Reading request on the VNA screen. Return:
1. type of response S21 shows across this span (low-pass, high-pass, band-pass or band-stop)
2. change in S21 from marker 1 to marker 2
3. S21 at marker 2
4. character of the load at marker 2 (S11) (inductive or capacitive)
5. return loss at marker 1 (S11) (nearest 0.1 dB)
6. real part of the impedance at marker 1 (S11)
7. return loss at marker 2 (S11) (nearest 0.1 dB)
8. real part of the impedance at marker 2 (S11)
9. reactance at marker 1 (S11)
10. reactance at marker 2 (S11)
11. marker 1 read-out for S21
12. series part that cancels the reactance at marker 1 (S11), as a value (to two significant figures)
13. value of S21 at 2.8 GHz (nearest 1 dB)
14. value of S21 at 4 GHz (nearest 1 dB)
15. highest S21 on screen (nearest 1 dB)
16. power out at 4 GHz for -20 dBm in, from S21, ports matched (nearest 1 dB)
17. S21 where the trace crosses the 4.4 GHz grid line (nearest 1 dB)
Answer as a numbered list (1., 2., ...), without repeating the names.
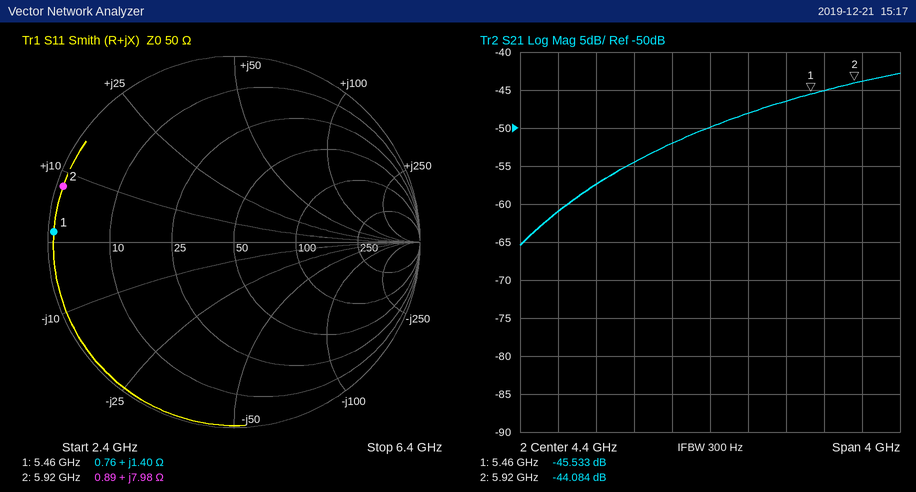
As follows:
1. high-pass
2. 1.449 dB
3. -44.084 dB
4. inductive
5. 0.3 dB
6. 0.76 Ω
7. 0.3 dB
8. 0.89 Ω
9. +1.40 Ω
10. +7.98 Ω
11. -45.533 dB
12. 21 pF
13. -61 dB
14. -52 dB
15. -43 dB
16. -72 dBm
17. -50 dB
